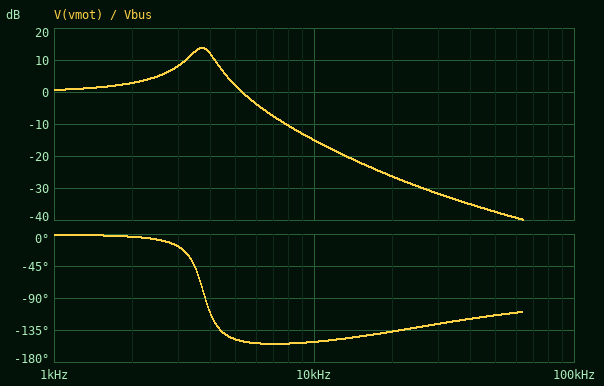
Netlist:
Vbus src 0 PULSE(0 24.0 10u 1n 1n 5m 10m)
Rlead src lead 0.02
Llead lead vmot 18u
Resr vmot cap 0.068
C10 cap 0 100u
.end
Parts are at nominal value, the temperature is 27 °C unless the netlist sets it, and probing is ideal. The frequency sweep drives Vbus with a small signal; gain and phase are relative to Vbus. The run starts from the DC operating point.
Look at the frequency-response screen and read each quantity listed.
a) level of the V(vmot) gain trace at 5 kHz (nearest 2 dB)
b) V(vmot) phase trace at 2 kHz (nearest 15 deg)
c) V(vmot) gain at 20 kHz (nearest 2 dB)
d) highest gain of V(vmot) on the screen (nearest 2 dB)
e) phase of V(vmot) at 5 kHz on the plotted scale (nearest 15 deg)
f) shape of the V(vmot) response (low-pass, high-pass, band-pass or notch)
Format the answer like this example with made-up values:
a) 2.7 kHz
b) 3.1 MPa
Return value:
a) 2 dB
b) 0 deg
c) -26 dB
d) 14 dB
e) -150 deg
f) low-pass
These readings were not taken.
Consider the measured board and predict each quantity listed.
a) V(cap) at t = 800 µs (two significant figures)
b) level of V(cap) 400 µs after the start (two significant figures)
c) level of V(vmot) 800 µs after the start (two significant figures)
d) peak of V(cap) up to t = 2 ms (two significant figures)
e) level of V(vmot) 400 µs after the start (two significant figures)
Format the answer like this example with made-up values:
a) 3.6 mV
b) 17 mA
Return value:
a) 21 V
b) 33 V
c) 21 V
d) 41 V
e) 33 V
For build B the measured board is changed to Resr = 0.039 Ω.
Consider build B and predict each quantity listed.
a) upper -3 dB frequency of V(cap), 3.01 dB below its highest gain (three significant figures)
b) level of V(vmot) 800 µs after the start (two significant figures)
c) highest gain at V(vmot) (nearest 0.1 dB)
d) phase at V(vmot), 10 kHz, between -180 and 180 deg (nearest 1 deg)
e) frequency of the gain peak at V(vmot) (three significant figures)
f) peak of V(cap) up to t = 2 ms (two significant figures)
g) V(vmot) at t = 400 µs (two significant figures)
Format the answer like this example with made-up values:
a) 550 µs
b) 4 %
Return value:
a) 3.99 kHz
b) 18 V
c) 17.2 dB
d) -163 deg
e) 3.73 kHz
f) 43 V
g) 36 V
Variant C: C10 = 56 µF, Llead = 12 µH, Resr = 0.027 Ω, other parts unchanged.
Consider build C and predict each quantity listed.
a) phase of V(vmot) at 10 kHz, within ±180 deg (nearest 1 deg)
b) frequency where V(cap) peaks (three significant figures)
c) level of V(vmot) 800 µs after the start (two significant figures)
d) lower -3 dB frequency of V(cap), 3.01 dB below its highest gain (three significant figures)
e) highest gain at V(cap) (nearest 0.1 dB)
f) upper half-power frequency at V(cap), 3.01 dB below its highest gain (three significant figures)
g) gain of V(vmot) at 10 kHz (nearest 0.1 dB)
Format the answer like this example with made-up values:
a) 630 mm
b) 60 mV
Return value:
a) -169 deg
b) 6.12 kHz
c) 21 V
d) 5.80 kHz
e) 19.9 dB
f) 6.43 kHz
g) -4.4 dB
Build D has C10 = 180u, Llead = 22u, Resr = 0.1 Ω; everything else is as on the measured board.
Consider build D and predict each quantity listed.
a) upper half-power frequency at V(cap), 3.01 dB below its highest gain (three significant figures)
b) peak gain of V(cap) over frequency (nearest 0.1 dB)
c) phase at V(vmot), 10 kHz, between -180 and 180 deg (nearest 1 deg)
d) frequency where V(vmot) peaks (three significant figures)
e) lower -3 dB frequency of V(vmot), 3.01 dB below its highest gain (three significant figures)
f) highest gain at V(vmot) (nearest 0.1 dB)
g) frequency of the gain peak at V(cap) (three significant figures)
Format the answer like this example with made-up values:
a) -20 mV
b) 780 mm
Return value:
a) 2.86 kHz
b) 9.4 dB
c) -126 deg
d) 2.46 kHz
e) 1.98 kHz
f) 9.7 dB
g) 2.45 kHz
